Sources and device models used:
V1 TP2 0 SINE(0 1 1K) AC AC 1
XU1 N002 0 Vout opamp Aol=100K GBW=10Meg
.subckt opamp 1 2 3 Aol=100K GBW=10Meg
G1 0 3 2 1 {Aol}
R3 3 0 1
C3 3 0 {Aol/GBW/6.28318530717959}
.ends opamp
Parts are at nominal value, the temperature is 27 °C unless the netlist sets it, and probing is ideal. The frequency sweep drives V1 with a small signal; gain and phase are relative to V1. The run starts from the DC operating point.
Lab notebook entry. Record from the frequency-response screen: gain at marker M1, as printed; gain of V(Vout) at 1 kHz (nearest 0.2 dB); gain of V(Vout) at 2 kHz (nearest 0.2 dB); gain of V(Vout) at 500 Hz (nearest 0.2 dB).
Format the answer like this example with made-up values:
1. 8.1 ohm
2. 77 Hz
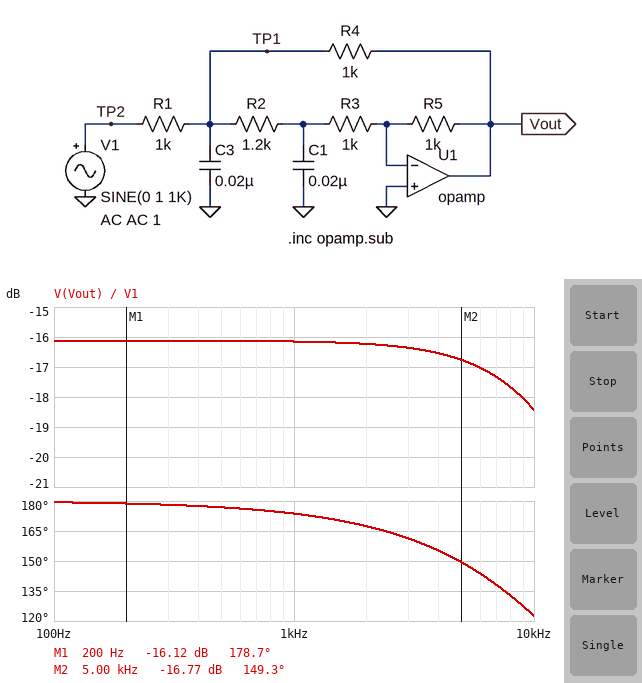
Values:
1. -16.12 dB
2. -16.2 dB
3. -16.2 dB
4. -16.2 dB
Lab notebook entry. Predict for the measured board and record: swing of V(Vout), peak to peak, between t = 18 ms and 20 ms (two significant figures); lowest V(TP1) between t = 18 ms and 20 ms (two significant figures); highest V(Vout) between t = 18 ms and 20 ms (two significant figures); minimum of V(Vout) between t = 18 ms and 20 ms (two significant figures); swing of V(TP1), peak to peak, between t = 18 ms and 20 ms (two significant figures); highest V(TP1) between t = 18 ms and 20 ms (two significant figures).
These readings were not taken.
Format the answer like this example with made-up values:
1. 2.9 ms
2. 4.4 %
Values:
1. 310 mV
2. -340 mV
3. 160 mV
4. -160 mV
5. 690 mV
6. 340 mV
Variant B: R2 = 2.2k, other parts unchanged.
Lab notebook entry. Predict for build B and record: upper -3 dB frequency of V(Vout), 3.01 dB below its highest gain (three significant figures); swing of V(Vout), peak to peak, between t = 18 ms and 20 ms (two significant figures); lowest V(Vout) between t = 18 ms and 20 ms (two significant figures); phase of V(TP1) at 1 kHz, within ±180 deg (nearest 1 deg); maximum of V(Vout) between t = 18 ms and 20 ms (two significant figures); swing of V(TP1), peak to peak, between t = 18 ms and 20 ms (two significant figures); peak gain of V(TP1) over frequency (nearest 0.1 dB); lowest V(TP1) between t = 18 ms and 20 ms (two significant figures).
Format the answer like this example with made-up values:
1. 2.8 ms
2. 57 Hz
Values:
1. 10.0 kHz
2. 240 mV
3. -120 mV
4. -2 deg
5. 120 mV
6. 760 mV
7. -8.4 dB
8. -380 mV
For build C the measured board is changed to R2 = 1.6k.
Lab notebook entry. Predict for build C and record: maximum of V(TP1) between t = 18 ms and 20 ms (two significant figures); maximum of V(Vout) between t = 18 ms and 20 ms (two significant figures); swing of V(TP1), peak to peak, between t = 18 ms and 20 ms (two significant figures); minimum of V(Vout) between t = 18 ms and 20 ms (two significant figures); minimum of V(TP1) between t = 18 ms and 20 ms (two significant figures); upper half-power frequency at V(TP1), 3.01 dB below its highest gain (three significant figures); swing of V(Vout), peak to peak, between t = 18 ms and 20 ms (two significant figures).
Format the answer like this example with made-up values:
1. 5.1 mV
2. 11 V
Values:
1. 360 mV
2. 140 mV
3. 720 mV
4. -140 mV
5. -360 mV
6. 23.4 kHz
7. 280 mV
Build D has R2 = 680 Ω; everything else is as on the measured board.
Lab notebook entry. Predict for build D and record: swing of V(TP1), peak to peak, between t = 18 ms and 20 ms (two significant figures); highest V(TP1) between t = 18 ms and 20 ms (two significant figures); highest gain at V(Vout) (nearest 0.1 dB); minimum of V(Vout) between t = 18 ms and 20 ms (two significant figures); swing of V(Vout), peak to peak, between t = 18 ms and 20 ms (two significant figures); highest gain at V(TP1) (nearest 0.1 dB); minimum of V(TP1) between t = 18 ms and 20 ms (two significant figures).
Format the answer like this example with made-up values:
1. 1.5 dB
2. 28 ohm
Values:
1. 630 mV
2. 310 mV
3. -14.6 dB
4. -190 mV
5. 370 mV
6. -10.1 dB
7. -310 mV
